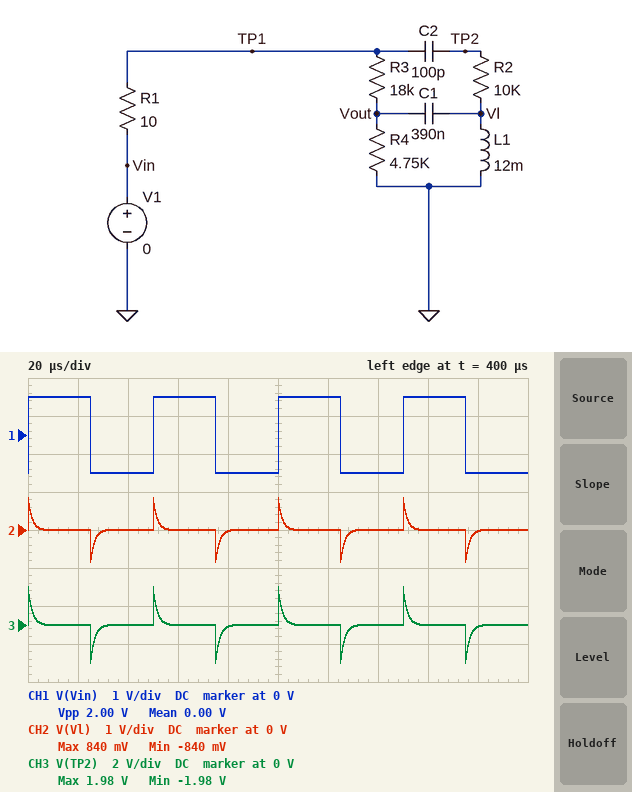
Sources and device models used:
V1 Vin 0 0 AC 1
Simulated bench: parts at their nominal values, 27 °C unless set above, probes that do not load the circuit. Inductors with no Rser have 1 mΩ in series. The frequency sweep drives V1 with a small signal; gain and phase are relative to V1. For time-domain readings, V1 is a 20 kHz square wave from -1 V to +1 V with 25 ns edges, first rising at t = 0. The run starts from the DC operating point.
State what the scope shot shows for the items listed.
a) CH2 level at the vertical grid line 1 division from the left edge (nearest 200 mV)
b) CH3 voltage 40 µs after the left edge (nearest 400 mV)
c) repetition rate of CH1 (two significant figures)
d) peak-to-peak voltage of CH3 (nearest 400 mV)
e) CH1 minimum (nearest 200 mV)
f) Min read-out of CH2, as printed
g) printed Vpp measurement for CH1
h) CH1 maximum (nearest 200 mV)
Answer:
0 V
0 V
20 kHz
4.0 V
-1.0 V
-840 mV
2.00 V
1.0 V
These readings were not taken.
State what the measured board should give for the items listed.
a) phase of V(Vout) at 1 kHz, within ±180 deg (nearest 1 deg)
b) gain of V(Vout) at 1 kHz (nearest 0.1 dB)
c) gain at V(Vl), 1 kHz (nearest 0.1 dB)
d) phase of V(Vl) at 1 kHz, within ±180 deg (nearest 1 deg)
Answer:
-85 deg
-34.7 dB
-47.6 dB
96 deg
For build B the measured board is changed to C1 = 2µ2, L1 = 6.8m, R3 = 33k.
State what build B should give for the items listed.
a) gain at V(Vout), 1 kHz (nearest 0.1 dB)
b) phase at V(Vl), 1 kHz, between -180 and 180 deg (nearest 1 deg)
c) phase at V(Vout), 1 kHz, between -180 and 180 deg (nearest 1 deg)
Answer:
-60.9 dB
92 deg
-91 deg
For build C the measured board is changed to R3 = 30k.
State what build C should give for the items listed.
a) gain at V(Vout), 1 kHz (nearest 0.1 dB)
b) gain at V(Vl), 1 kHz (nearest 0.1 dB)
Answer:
-39.1 dB
-52.0 dB
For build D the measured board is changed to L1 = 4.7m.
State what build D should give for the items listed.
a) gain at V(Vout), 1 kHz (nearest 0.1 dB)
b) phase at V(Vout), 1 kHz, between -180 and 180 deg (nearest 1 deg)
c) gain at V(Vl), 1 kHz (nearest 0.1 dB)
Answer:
-33.6 dB
-84 deg
-55.7 dB
